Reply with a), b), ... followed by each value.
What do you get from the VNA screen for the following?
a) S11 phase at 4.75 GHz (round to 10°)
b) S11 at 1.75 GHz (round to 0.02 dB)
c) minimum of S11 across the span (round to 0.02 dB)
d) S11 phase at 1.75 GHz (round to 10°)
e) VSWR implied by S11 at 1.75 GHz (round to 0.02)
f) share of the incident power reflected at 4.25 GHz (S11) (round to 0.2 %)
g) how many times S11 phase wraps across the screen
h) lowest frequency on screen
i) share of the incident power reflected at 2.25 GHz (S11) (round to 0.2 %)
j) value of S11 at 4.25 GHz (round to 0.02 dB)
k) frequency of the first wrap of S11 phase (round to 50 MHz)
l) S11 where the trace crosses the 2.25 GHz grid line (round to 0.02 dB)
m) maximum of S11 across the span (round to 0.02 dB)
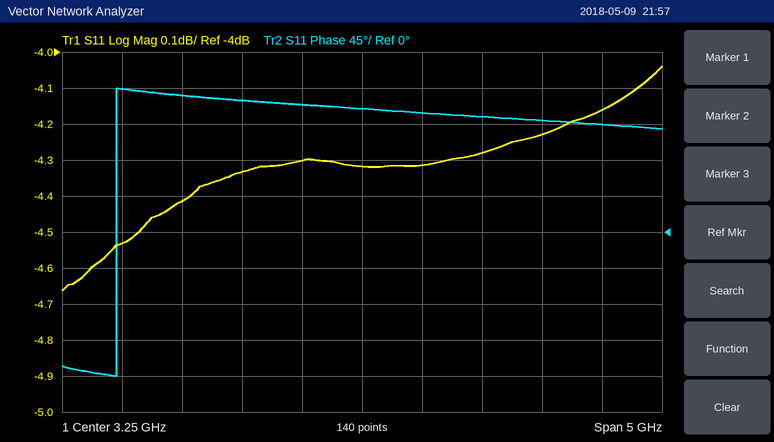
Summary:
a) 140°
b) -4.42 dB
c) -4.66 dB
d) 170°
e) 4.02
f) 37.4 %
g) 1
h) 750 MHz
i) 36.8 %
j) -4.28 dB
k) 1.20 GHz
l) -4.34 dB
m) -4.04 dB
